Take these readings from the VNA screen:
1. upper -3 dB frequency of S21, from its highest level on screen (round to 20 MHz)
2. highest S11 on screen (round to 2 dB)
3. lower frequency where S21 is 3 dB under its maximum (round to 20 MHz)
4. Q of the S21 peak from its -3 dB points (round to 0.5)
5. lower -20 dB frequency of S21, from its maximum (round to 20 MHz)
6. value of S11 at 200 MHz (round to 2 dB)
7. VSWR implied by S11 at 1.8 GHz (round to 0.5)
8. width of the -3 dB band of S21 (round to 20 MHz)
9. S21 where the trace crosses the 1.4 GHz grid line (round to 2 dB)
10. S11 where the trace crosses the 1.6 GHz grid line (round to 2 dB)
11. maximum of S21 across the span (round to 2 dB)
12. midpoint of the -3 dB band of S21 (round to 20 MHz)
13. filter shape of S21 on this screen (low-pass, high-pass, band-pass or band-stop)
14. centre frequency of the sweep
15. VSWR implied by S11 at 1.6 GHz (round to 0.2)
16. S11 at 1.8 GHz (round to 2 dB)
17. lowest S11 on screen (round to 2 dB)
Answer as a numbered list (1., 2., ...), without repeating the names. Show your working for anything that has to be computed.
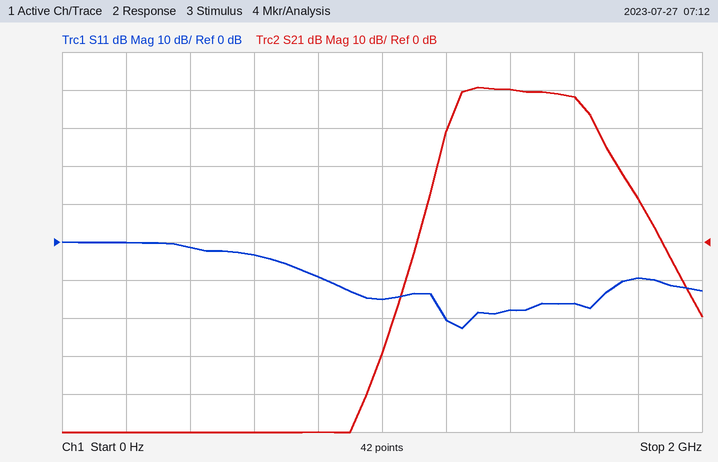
1. 1.60 GHz
2. 0 dB
3. 1.24 GHz
4. 1.42 GHz / 360 MHz ≈ 3.94, so 4.0 to the nearest 0.5
5. 1.18 GHz
6. 0 dB
7. |Γ| = 10^(-10/20) = 0.3162; VSWR = (1 + 0.3162)/(1 − 0.3162) ≈ 1.92, so 2.0 to the nearest 0.5
8. 1.60 GHz − 1.24 GHz = 360 MHz
9. 40 dB
10. -16 dB
11. 40 dB
12. 1.42 GHz
13. band-pass
14. 1 GHz
15. |Γ| = 10^(-16/20) = 0.1585; VSWR = (1 + 0.1585)/(1 − 0.1585) ≈ 1.4
16. -10 dB
17. -22 dB
